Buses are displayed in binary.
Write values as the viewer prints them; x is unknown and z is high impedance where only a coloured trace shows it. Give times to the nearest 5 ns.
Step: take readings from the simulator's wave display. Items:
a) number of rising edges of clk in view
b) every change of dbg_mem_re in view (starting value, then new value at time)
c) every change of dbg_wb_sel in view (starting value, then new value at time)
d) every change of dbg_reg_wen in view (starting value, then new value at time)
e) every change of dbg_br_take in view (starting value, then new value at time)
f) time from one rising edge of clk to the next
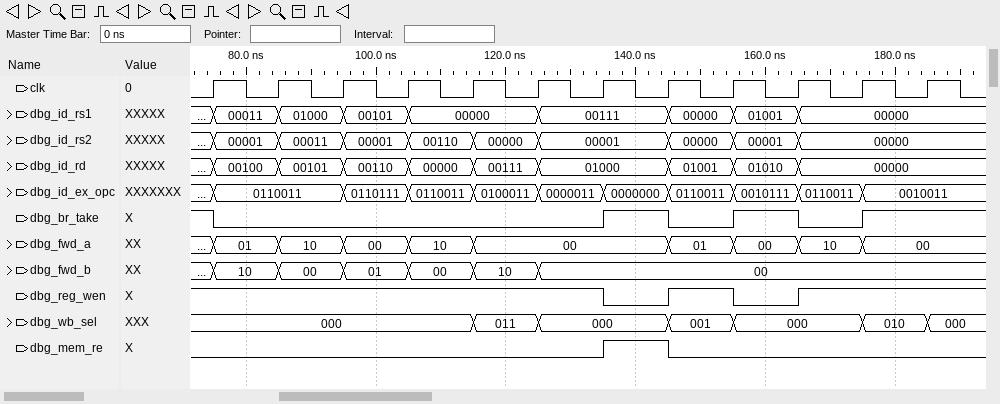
12
0, 1 at 135 ns, 0 at 145 ns
000, 011 at 115 ns, 000 at 125 ns, 001 at 145 ns, 000 at 155 ns, 010 at 175 ns, 000 at 185 ns
1, 0 at 135 ns, 1 at 145 ns, 0 at 155 ns, 1 at 165 ns
1, 0 at 75 ns, 1 at 135 ns, 0 at 145 ns, 1 at 155 ns, 0 at 165 ns, 1 at 175 ns
10 ns
